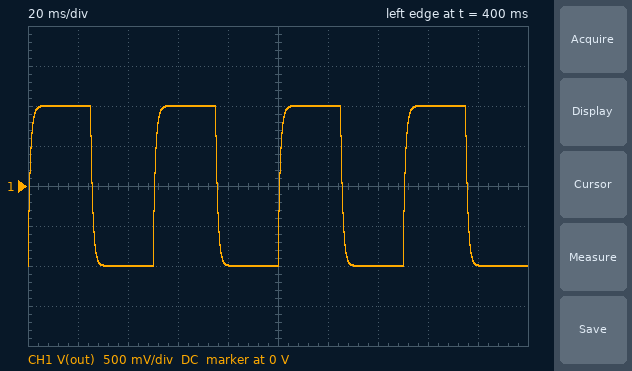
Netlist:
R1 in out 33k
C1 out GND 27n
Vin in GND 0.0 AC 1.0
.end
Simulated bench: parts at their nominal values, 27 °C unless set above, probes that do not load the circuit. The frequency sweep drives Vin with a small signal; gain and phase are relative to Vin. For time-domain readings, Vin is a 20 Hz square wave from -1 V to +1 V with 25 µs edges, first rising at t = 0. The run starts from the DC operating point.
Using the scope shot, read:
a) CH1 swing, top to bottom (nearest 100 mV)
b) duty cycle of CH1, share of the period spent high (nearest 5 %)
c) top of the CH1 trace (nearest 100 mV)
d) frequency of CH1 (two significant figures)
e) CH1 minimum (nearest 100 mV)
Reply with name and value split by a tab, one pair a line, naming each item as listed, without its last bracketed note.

CH1 swing, top to bottom	2.0 V
duty cycle of CH1, share of the period spent high	50 %
top of the CH1 trace	1.0 V
frequency of CH1	20 Hz
CH1 minimum	-1.0 V
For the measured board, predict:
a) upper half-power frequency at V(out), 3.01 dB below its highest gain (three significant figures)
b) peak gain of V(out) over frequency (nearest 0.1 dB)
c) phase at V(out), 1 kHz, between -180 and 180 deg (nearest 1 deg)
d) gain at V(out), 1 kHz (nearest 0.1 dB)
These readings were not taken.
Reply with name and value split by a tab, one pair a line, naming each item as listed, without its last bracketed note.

upper half-power frequency at V(out), 3.01 dB below its highest gain	179 Hz
peak gain of V(out) over frequency	0 dB
phase at V(out), 1 kHz, between -180 and 180 deg	-80 deg
gain at V(out), 1 kHz	-15.1 dB
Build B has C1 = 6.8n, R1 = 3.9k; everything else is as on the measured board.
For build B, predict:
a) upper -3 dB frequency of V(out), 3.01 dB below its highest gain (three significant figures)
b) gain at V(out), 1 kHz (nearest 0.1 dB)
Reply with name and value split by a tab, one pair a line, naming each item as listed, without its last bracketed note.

upper -3 dB frequency of V(out), 3.01 dB below its highest gain	6.00 kHz
gain at V(out), 1 kHz	-0.1 dB
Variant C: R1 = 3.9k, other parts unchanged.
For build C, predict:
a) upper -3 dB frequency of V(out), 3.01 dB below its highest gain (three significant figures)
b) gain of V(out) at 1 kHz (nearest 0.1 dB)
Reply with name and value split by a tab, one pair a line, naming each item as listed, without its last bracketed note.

upper -3 dB frequency of V(out), 3.01 dB below its highest gain	1.51 kHz
gain of V(out) at 1 kHz	-1.6 dB
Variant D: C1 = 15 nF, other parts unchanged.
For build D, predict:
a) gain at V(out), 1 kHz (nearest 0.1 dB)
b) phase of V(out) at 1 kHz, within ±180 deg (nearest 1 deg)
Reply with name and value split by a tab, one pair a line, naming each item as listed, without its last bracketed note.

gain at V(out), 1 kHz	-10.3 dB
phase of V(out) at 1 kHz, within ±180 deg	-72 deg
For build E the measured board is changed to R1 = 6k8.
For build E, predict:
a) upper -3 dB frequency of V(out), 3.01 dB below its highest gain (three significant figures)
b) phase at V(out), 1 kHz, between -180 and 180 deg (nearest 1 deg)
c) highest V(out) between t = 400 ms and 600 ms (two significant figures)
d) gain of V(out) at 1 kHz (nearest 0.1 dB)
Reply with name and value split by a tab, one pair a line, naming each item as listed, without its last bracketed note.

upper -3 dB frequency of V(out), 3.01 dB below its highest gain	867 Hz
phase at V(out), 1 kHz, between -180 and 180 deg	-49 deg
highest V(out) between t = 400 ms and 600 ms	1.0 V
gain of V(out) at 1 kHz	-3.7 dB
